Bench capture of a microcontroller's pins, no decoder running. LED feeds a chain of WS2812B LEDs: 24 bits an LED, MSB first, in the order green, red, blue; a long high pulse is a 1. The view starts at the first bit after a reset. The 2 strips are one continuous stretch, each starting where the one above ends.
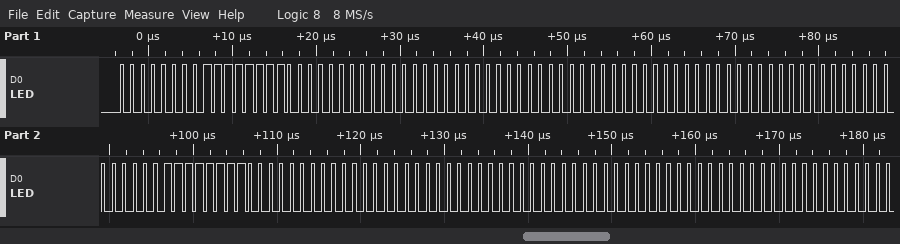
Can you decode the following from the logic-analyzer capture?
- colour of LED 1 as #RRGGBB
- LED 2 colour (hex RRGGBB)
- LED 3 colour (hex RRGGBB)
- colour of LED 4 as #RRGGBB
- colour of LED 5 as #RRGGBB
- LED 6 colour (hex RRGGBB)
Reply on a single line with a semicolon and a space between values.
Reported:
#FF0000; #000000; #000000; #FF0000; #000000; #000000
